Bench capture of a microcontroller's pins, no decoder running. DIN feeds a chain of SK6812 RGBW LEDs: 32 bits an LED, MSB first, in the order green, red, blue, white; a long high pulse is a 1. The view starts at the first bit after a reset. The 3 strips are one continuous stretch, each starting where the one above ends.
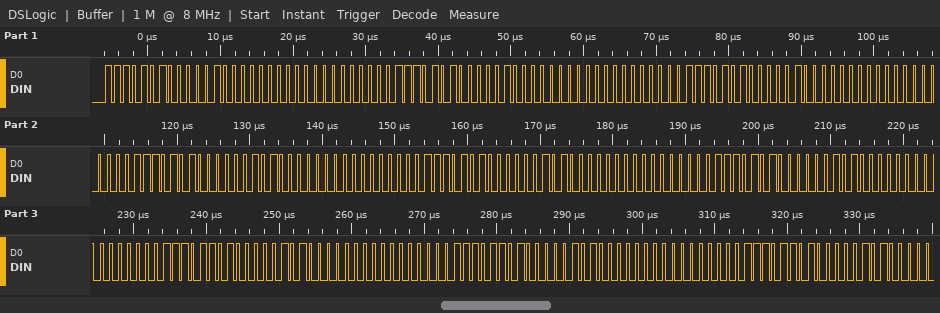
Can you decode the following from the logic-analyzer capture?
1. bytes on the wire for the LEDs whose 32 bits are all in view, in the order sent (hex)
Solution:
EA 08 00 00 EA 08 00 00 EA 08 00 00 EA 05 00 00 EA 05 00 00 EA 05 00 00 ED 05 00 00 ED 05 00 00
